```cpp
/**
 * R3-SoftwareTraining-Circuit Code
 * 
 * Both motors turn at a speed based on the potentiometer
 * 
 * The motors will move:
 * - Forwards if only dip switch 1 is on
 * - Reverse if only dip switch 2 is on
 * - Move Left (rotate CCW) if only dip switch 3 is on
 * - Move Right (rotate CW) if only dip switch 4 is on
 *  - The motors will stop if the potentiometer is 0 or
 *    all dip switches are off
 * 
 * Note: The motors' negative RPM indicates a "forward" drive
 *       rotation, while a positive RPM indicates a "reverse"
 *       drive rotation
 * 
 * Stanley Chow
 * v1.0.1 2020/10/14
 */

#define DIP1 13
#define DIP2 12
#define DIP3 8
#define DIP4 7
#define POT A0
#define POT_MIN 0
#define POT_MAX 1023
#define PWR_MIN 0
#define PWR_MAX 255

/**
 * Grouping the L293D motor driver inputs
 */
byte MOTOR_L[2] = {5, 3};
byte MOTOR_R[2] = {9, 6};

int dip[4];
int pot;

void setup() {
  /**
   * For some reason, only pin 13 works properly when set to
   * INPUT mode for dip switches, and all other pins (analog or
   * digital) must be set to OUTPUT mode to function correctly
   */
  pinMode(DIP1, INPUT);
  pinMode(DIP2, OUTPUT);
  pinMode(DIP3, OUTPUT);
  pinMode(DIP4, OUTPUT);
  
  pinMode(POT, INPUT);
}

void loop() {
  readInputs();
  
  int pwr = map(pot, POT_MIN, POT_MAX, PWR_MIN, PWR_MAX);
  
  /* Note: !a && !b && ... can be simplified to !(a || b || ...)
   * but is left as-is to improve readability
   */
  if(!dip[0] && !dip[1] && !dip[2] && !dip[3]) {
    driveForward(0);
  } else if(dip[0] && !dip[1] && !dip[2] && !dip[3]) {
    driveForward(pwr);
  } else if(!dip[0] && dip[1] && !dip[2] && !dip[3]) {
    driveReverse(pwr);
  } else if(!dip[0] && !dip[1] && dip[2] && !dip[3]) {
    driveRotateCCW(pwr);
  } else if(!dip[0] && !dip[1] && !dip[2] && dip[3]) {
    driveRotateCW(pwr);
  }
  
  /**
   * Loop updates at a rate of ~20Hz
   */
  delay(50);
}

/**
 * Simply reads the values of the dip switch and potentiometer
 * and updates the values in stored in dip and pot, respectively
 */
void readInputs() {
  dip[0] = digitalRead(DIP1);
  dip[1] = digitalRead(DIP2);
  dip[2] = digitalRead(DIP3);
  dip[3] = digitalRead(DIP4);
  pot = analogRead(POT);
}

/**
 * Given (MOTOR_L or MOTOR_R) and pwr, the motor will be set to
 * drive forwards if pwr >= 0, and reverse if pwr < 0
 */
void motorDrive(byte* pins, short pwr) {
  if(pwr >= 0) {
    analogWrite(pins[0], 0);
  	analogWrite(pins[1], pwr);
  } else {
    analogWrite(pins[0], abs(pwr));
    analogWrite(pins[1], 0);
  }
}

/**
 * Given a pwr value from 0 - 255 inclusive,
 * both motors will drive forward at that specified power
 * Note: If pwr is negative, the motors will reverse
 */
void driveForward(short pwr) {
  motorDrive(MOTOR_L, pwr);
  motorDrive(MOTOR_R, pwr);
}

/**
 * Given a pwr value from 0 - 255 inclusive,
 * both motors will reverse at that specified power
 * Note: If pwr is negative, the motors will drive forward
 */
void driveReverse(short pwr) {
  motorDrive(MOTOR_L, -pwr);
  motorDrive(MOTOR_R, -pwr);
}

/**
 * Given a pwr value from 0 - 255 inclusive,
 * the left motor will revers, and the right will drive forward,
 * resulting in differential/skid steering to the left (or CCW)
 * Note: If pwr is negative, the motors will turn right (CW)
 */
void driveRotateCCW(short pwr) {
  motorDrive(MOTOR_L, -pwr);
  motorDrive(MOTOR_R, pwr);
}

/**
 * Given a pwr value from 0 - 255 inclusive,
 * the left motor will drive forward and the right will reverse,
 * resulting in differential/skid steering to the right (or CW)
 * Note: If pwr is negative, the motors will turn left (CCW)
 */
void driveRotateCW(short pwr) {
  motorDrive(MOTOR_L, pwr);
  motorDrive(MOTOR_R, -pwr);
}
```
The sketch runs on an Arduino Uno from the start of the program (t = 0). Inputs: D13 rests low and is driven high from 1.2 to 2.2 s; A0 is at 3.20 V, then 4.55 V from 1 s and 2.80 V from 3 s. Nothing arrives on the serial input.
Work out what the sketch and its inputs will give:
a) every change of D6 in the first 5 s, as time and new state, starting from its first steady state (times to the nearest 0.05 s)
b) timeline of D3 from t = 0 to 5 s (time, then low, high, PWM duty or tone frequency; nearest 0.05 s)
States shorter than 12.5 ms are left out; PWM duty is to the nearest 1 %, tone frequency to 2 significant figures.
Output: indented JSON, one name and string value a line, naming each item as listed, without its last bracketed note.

{
  "every change of D6 in the first 5 s, as time and new state, starting from its first steady state": "0 s low; 1.2 s PWM 91 %; 2.2 s low",
  "timeline of D3 from t = 0 to 5 s": "0 s low; 1.2 s PWM 91 %; 2.2 s low"
}
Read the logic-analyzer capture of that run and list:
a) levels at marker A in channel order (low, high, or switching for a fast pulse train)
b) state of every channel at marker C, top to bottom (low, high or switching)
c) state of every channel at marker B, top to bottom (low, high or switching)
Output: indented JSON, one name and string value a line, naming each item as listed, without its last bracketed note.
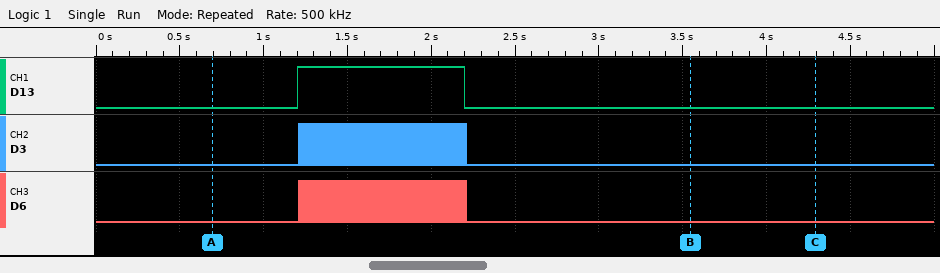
{
  "levels at marker A in channel order": "D13 low, D3 low, D6 low",
  "state of every channel at marker C, top to bottom": "D13 low, D3 low, D6 low",
  "state of every channel at marker B, top to bottom": "D13 low, D3 low, D6 low"
}
